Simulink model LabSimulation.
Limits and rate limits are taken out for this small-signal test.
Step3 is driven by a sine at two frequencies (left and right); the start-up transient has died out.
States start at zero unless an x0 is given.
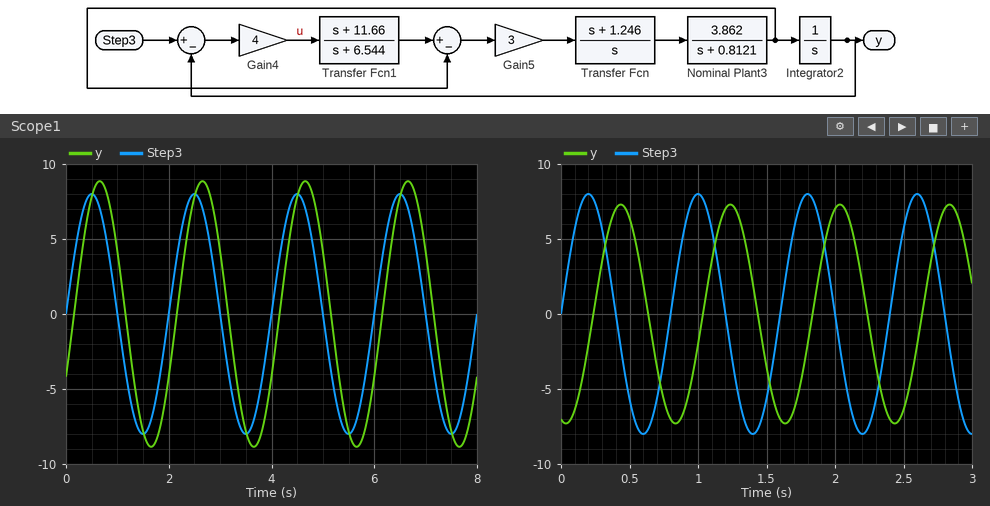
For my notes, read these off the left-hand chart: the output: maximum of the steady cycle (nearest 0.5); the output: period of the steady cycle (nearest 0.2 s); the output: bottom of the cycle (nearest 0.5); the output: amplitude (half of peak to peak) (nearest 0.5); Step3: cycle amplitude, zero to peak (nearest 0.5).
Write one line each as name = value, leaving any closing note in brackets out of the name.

the output: maximum of the steady cycle = 9.0
the output: period of the steady cycle = 2.0 s
the output: bottom of the cycle = -9.0
the output: amplitude (half of peak to peak) = 9.0
Step3: cycle amplitude, zero to peak = 8.0
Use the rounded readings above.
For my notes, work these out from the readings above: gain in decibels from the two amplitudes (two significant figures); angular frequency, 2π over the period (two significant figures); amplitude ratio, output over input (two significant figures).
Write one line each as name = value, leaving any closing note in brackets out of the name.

gain in decibels from the two amplitudes = 1.0 dB
angular frequency, 2π over the period = 3.1 rad/s
amplitude ratio, output over input = 1.1
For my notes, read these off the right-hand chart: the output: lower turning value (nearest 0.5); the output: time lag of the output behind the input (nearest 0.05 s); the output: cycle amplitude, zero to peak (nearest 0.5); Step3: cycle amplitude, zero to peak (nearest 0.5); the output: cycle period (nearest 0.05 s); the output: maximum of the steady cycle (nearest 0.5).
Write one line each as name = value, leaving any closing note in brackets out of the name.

the output: lower turning value = -7.5
the output: time lag of the output behind the input = 0.25 s
the output: cycle amplitude, zero to peak = 7.5
Step3: cycle amplitude, zero to peak = 8.0
the output: cycle period = 0.80 s
the output: maximum of the steady cycle = 7.5
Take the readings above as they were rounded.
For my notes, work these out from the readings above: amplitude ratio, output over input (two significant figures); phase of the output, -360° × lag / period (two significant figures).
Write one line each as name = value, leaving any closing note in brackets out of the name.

amplitude ratio, output over input = 0.94
phase of the output, -360° × lag / period = -110°
